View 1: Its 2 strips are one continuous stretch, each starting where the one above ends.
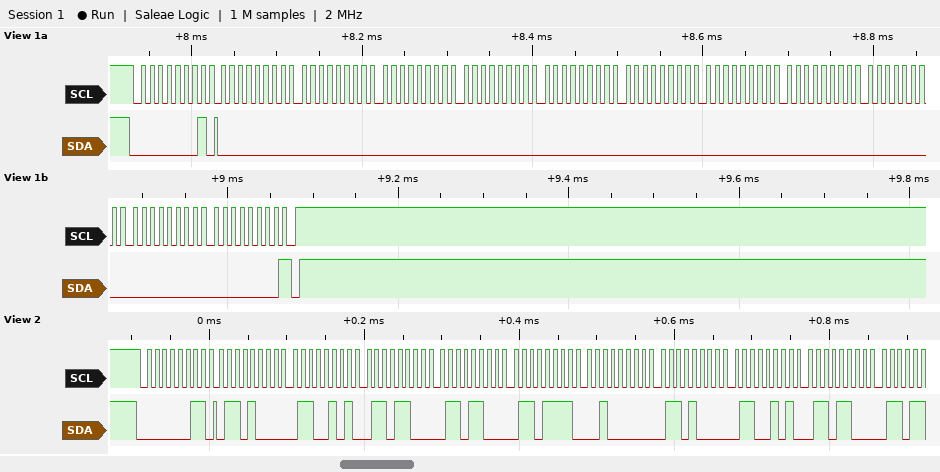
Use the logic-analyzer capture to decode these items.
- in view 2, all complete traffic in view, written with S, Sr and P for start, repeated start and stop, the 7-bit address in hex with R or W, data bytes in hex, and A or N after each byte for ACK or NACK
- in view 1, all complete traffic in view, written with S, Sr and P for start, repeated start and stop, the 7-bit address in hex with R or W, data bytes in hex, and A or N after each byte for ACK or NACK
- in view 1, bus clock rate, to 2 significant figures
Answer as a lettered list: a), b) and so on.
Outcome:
a) S 01R A 68 A 65 A 6C A 6C A 6F A 20 A 68 A 65 A 6C A
b) S 00R A 00 A 00 A 00 A 00 A 00 A 00 A 00 A 00 A 00 A 00 A 00 N P
c) 100 kHz
